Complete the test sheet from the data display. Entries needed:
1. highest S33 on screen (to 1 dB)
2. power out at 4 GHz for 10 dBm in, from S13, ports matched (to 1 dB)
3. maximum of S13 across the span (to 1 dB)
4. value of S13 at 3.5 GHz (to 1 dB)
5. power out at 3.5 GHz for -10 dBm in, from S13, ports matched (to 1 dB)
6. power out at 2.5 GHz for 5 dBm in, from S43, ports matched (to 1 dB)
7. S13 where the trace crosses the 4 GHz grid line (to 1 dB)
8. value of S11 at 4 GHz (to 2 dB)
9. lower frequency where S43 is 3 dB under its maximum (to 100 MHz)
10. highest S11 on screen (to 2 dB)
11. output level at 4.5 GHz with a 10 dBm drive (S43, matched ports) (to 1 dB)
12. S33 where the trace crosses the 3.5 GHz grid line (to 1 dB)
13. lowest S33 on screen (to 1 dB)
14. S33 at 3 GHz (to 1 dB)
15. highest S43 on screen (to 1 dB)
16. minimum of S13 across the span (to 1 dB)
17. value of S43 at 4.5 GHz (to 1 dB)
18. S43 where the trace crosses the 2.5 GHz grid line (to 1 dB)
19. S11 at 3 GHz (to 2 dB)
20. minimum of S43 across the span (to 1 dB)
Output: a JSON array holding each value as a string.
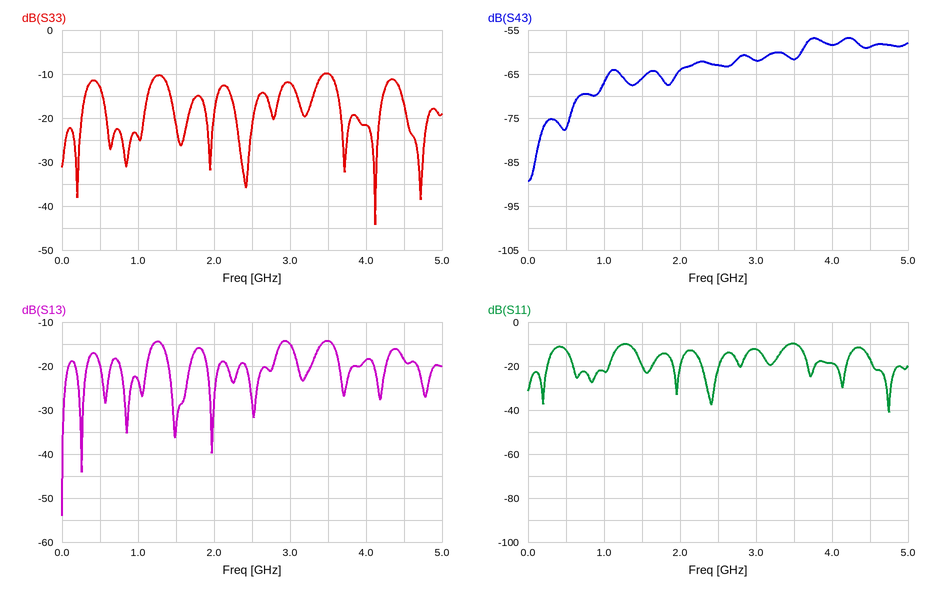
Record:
["-10 dB", "-9 dBm", "-14 dB", "-14 dB", "-24 dBm", "-58 dBm", "-19 dB", "-18 dB", "3.6 GHz", "-10 dB", "-49 dBm", "-10 dB", "-44 dB", "-12 dB", "-57 dB", "-54 dB", "-59 dB", "-63 dB", "-12 dB", "-89 dB"]
